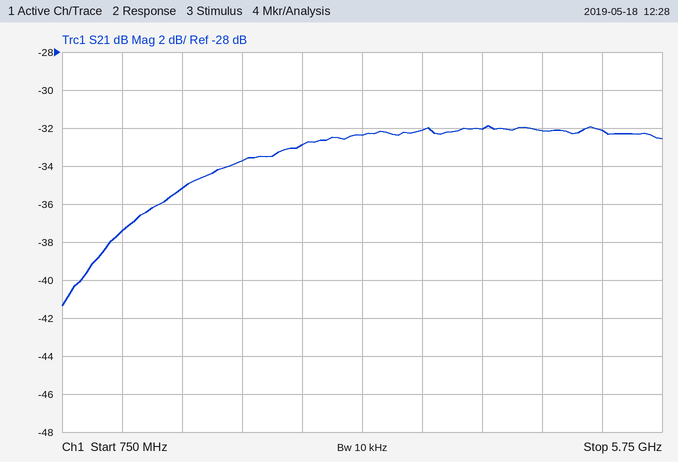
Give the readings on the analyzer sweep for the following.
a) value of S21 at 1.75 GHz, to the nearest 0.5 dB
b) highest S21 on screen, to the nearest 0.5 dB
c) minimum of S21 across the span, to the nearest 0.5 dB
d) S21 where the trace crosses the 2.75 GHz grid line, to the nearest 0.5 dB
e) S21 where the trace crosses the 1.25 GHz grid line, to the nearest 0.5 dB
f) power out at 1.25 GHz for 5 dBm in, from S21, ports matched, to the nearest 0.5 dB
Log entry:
-35.0 dB
-32.0 dB
-41.5 dB
-33.0 dB
-37.5 dB
-32.5 dBm
